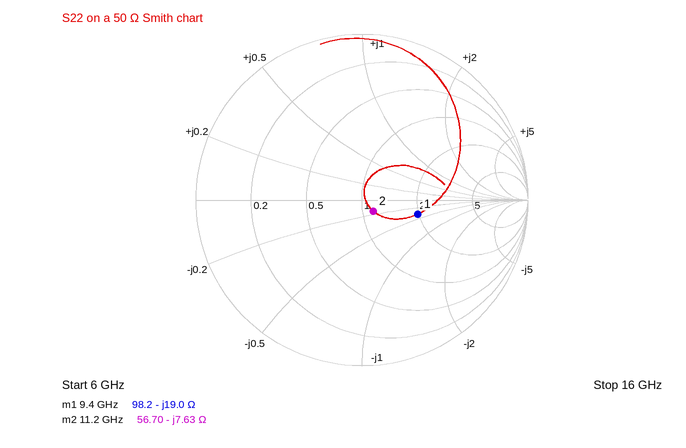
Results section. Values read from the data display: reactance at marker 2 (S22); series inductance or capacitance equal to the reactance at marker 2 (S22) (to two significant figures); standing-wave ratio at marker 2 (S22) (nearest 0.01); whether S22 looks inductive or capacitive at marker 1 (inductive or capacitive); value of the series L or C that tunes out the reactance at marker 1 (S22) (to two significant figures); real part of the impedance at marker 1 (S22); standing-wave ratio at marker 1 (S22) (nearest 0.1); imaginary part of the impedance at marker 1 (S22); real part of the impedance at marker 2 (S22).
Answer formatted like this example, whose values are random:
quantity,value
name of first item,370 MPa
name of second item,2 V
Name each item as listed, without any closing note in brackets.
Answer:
quantity,value
reactance at marker 2,-7.63 Ω
series inductance or capacitance equal to the reactance at marker 2 (S22),1.9 pF
standing-wave ratio at marker 2 (S22),1.21
whether S22 looks inductive or capacitive at marker 1,capacitive
value of the series L or C that tunes out the reactance at marker 1 (S22),320 pH
real part of the impedance at marker 1,98.2 Ω
standing-wave ratio at marker 1 (S22),2.1
imaginary part of the impedance at marker 1,-19.0 Ω
real part of the impedance at marker 2,56.70 Ω
